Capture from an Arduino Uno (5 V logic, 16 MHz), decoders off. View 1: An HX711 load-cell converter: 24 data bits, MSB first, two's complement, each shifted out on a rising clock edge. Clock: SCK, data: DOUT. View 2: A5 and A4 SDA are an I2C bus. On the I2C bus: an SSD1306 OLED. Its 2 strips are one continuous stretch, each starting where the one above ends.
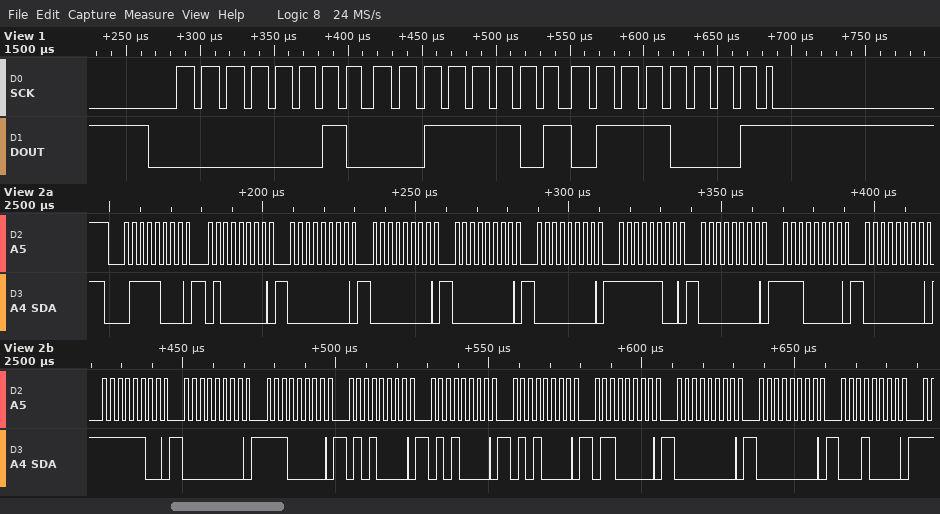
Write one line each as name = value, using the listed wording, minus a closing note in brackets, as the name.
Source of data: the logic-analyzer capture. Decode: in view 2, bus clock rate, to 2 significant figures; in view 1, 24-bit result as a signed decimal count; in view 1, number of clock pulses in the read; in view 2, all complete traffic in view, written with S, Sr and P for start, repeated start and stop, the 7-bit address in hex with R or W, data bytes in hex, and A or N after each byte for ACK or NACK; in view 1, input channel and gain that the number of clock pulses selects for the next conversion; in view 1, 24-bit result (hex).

in view 2, bus clock rate, to 2 significant figures = 400 kHz
in view 1, 24-bit result as a signed decimal count = 146801
in view 1, number of clock pulses in the read = 25
in view 2, all complete traffic in view, written with S, Sr and P for start, repeated start and stop, the 7-bit address in hex with R or W, data bytes in hex, and A or N after each byte for ACK or NACK = S 3CW A 40 A 00 A 00 A 00 A 00 A FC A 00 A E0 A 00 A FC A 00 A E0 A 50 A 50 A 50 A 60 A 00 A 00 A 10 A
in view 1, input channel and gain that the number of clock pulses selects for the next conversion = channel A, gain 128
in view 1, 24-bit result = 0x023D71
